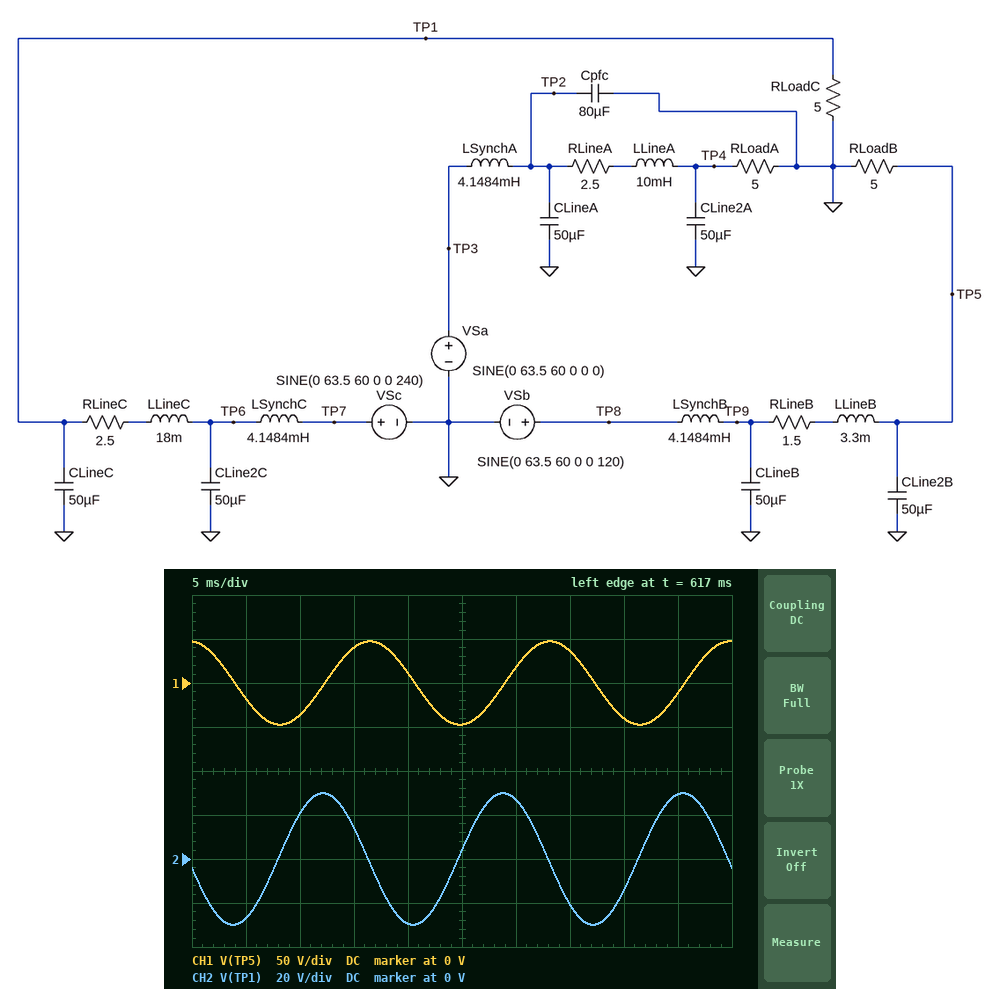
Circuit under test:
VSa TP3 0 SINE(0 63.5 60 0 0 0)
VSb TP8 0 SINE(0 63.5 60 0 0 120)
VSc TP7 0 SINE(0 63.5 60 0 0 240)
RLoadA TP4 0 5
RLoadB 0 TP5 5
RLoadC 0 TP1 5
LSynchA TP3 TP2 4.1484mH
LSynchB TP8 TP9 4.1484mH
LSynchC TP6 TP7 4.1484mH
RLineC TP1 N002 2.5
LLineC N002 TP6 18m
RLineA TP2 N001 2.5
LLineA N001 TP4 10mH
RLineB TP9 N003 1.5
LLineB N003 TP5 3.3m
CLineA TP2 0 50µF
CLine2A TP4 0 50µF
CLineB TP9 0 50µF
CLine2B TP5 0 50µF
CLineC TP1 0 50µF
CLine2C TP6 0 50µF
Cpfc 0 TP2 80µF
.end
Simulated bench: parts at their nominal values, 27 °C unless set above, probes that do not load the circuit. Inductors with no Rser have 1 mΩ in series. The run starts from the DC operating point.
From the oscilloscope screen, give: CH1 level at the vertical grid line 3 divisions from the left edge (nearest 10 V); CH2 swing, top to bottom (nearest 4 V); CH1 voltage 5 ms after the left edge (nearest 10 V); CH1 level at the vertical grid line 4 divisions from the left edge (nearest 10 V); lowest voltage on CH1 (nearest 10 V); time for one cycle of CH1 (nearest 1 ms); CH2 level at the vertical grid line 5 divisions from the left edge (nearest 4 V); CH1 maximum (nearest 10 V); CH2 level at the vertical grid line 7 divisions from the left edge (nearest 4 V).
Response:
40 V
60 V
-20 V
10 V
-50 V
17 ms
4 V
50 V
-20 V
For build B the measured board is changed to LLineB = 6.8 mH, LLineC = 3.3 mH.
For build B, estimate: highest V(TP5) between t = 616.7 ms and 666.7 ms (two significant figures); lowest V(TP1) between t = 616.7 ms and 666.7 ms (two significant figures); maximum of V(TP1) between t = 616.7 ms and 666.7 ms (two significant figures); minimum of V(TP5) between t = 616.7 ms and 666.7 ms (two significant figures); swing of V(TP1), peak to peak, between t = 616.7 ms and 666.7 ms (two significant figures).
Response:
44 V
-42 V
42 V
-44 V
83 V
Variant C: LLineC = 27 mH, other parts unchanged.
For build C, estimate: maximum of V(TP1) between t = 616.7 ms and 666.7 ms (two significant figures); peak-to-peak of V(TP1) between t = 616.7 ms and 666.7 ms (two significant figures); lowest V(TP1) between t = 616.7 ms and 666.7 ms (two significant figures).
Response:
24 V
48 V
-24 V
